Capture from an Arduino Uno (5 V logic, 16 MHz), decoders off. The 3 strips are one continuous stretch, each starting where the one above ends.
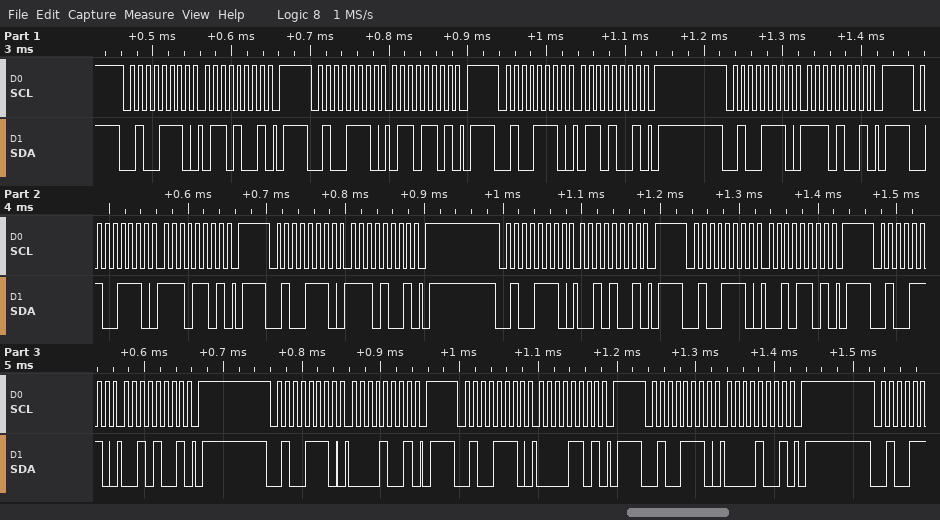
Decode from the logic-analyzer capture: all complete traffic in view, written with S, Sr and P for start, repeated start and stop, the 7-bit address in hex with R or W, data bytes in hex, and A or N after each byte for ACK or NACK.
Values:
S 27W A 69 A P S 27W A 6D A P S 27W A 69 A P S 27W A E9 A P S 27W A ED A P S 27W A E9 A P S 27W A 29 A P S 27W A 2D A P S 27W A 29 A P S 27W A 09 A P S 27W A 0D A P S 27W A 09 A P
